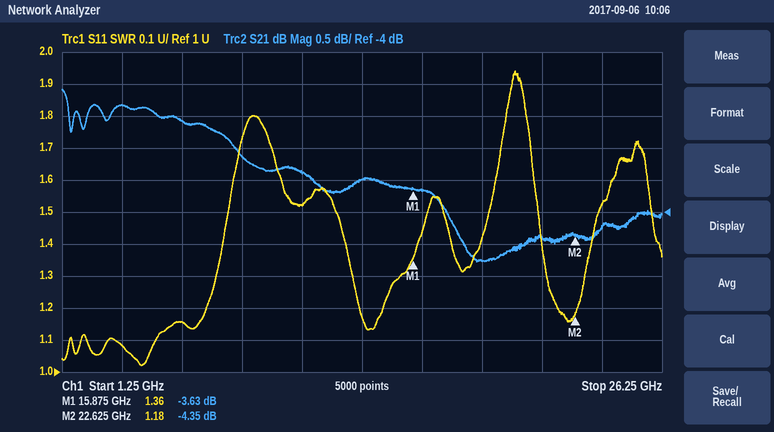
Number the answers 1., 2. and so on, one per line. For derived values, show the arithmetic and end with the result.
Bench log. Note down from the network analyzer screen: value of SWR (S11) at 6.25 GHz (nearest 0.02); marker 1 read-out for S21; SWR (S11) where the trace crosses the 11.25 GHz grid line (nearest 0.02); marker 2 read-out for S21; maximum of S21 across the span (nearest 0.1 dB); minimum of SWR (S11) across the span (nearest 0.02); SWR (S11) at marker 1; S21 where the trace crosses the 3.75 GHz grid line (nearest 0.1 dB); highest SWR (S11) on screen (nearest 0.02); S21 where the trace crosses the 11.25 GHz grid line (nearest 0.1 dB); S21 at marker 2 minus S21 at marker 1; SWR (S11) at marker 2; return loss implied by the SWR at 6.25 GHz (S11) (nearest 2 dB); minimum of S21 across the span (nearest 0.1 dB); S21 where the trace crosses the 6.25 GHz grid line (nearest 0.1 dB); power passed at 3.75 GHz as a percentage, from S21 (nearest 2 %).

1. 1.16
2. -3.63 dB
3. 1.52
4. -4.35 dB
5. -2.1 dB
6. 1.02
7. 1.36
8. -2.3 dB
9. 1.94
10. -3.4 dB
11. -4.35 − (-3.63) = -0.72 dB
12. 1.18
13. −20 log10((1.16 − 1)/(1.16 + 1)) ≈ 22.6 dB, so 22 dB to the nearest 2 dB
14. -4.8 dB
15. -2.6 dB
16. 10^(-2.3/10) ≈ 58.9 %, so 58 % to the nearest 2 %
